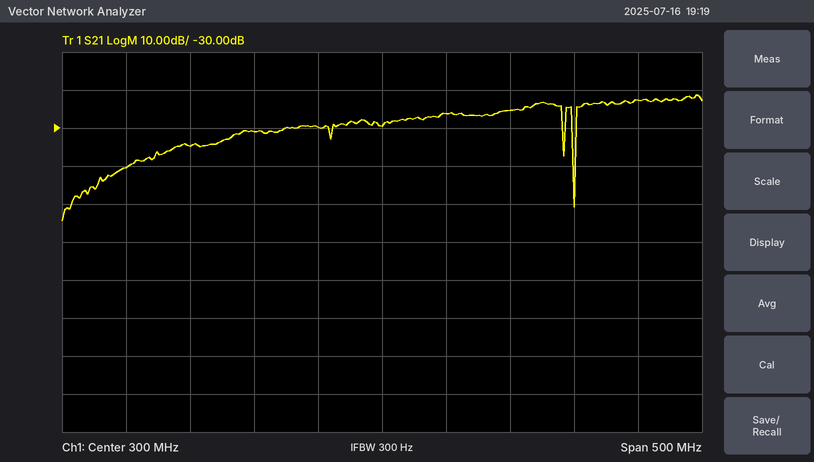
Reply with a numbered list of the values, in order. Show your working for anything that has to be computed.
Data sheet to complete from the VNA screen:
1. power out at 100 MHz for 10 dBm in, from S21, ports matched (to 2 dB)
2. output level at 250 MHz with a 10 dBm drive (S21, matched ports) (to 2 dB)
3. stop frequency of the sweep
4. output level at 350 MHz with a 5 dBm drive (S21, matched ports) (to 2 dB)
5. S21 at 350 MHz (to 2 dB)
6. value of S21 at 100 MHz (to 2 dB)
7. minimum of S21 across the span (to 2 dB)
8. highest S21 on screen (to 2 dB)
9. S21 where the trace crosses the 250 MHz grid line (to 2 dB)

1. 10 dBm + (-40 dB) = -30 dBm
2. 10 dBm + (-30 dB) = -20 dBm
3. 550 MHz
4. 5 dBm + (-26 dB) = -22 dBm
5. -26 dB
6. -40 dB
7. -54 dB
8. -22 dB
9. -30 dB
